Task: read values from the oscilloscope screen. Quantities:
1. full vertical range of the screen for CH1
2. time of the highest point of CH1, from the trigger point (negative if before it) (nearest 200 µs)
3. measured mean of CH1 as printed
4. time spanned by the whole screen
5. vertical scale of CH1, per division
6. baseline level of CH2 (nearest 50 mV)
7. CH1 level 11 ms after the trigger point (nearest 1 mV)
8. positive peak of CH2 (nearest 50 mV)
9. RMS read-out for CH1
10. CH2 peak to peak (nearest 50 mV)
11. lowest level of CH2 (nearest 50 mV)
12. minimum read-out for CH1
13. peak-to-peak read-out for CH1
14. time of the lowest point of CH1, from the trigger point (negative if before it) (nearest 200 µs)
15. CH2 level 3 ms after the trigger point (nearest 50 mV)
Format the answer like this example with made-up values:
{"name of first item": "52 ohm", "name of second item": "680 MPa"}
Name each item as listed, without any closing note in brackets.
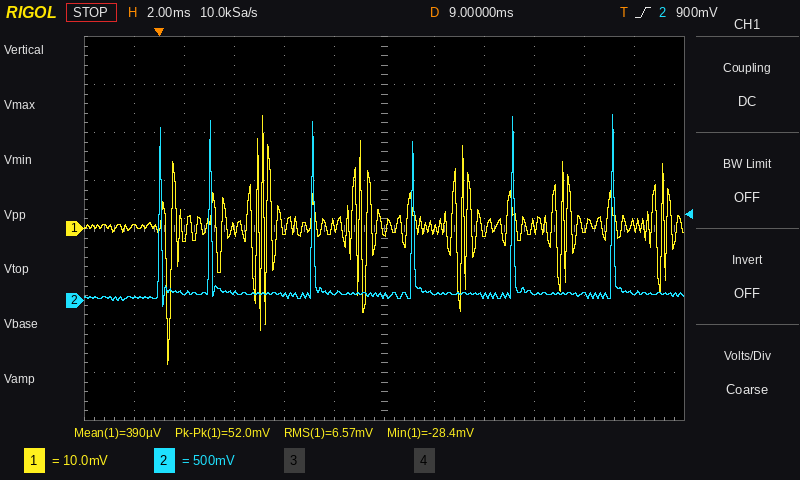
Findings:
{"full vertical range of the screen for CH1": "80 mV", "time of the highest point of CH1, from the trigger point (negative if before it)": "+4.2 ms", "measured mean of CH1 as printed": "390 µV", "time spanned by the whole screen": "24 ms", "vertical scale of CH1, per division": "10 mV", "baseline level of CH2": "50 mV", "CH1 level 11 ms after the trigger point": "0 mV", "positive peak of CH2": "1.95 V", "RMS read-out for CH1": "6.57 mV", "CH2 peak to peak": "2.00 V", "lowest level of CH2": "-50 mV", "minimum read-out for CH1": "-28.4 mV", "peak-to-peak read-out for CH1": "52.0 mV", "time of the lowest point of CH1, from the trigger point (negative if before it)": "+400 µs", "CH2 level 3 ms after the trigger point": "100 mV"}
